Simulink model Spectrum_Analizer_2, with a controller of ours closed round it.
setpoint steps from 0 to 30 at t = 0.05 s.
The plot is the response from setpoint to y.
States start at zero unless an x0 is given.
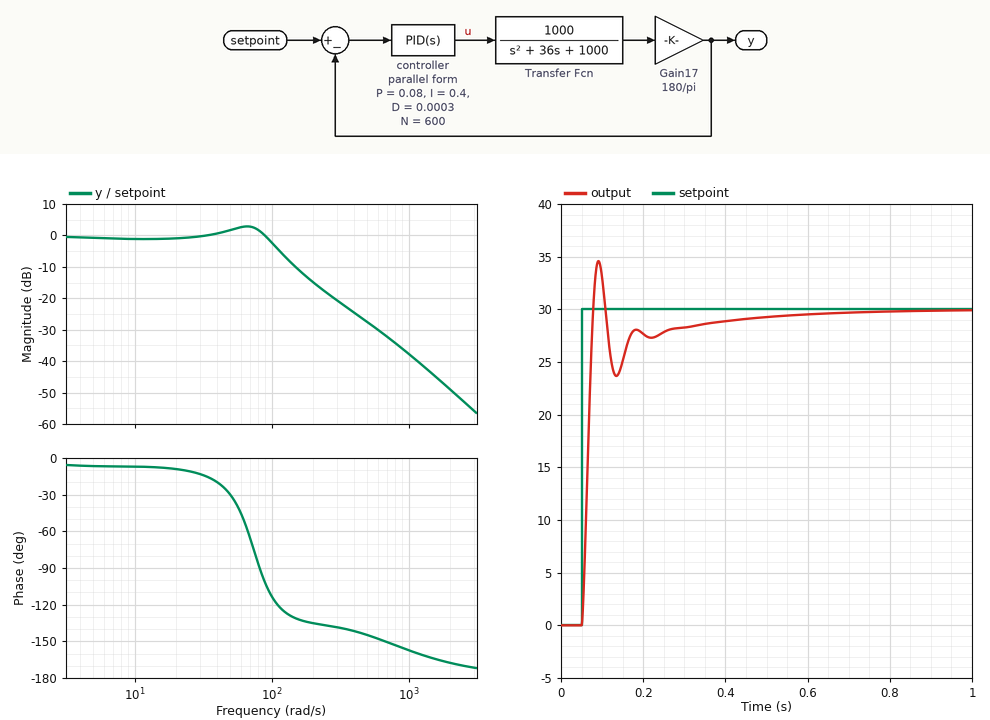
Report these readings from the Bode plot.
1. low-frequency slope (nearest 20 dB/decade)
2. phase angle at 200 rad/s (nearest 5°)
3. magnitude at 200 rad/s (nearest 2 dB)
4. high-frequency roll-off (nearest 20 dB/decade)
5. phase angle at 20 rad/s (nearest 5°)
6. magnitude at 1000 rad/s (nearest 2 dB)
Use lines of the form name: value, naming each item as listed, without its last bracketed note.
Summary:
low-frequency slope: 0 dB/decade
phase angle at 200 rad/s: -135°
magnitude at 200 rad/s: -14 dB
high-frequency roll-off: -40 dB/decade
phase angle at 20 rad/s: -10°
magnitude at 1000 rad/s: -38 dB
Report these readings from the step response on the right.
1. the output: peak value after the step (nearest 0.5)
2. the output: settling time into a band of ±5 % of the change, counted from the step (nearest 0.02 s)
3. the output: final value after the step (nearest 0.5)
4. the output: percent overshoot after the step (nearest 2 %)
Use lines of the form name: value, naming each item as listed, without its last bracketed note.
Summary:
the output: peak value after the step: 34.5
the output: settling time into a band of ±5 % of the change, counted from the step: 0.28 s
the output: final value after the step: 30.0
the output: percent overshoot after the step: 16 %
